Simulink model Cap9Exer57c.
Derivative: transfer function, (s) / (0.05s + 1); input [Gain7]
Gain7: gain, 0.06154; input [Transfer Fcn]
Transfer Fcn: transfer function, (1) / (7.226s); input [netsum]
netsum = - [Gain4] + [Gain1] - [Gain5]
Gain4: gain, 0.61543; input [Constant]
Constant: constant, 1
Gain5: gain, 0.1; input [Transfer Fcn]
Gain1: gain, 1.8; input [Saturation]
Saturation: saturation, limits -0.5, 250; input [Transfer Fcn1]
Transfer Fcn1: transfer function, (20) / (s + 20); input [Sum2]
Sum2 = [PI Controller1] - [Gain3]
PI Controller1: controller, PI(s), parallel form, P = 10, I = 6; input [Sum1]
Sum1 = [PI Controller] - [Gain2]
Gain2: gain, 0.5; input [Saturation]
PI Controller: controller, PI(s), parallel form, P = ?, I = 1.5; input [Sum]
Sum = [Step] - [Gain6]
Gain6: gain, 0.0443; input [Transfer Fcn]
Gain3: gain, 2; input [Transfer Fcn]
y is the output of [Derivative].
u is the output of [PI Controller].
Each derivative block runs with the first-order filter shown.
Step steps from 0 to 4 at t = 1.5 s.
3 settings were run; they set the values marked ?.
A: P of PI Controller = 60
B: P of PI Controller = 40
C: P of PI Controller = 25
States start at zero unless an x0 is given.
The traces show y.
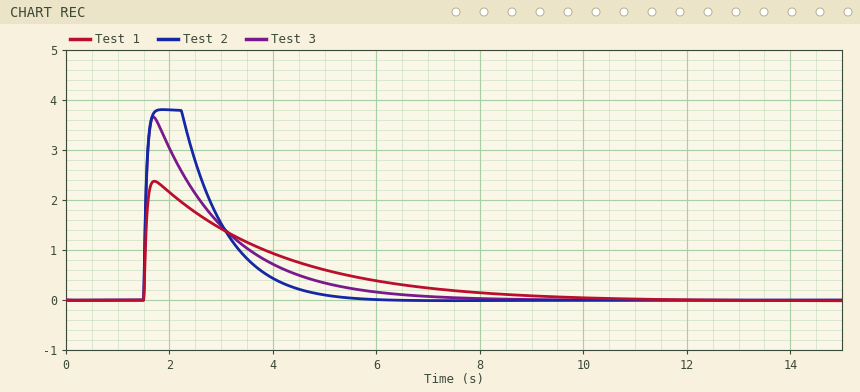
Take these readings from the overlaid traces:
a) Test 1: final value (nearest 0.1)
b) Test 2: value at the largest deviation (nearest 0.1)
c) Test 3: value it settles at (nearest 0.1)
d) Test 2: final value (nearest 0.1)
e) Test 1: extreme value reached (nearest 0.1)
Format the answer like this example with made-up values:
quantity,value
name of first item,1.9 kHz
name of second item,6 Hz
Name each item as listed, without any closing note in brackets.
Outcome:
quantity,value
Test 1: final value,0.0
Test 2: value at the largest deviation,3.8
Test 3: value it settles at,0.0
Test 2: final value,0.0
Test 1: extreme value reached,2.4
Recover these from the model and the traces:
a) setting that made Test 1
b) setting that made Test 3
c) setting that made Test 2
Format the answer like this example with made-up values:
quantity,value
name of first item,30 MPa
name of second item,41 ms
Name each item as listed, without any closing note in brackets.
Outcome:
quantity,value
setting that made Test 1,C
setting that made Test 3,B
setting that made Test 2,A
